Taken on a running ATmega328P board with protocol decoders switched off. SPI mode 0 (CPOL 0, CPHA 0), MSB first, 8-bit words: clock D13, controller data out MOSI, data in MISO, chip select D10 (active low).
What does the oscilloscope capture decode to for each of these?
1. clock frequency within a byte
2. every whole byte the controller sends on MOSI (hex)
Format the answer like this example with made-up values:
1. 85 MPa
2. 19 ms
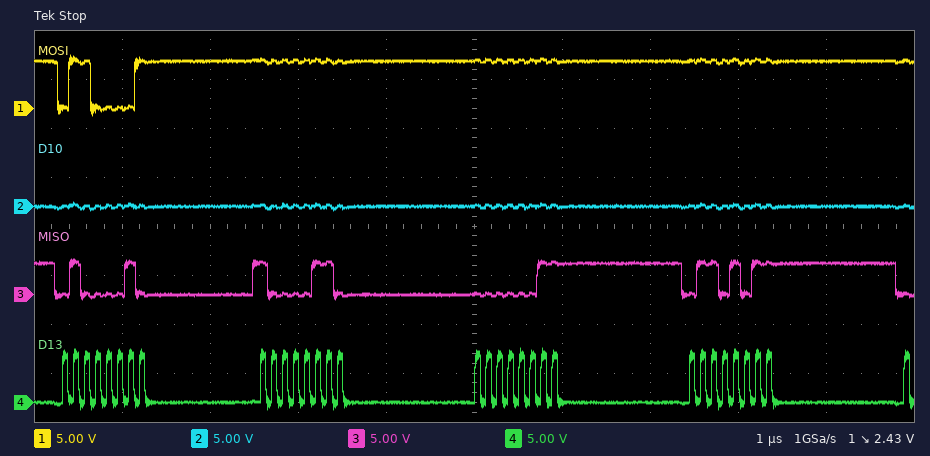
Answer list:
1. 8 MHz
2. 61 FF FF FF
